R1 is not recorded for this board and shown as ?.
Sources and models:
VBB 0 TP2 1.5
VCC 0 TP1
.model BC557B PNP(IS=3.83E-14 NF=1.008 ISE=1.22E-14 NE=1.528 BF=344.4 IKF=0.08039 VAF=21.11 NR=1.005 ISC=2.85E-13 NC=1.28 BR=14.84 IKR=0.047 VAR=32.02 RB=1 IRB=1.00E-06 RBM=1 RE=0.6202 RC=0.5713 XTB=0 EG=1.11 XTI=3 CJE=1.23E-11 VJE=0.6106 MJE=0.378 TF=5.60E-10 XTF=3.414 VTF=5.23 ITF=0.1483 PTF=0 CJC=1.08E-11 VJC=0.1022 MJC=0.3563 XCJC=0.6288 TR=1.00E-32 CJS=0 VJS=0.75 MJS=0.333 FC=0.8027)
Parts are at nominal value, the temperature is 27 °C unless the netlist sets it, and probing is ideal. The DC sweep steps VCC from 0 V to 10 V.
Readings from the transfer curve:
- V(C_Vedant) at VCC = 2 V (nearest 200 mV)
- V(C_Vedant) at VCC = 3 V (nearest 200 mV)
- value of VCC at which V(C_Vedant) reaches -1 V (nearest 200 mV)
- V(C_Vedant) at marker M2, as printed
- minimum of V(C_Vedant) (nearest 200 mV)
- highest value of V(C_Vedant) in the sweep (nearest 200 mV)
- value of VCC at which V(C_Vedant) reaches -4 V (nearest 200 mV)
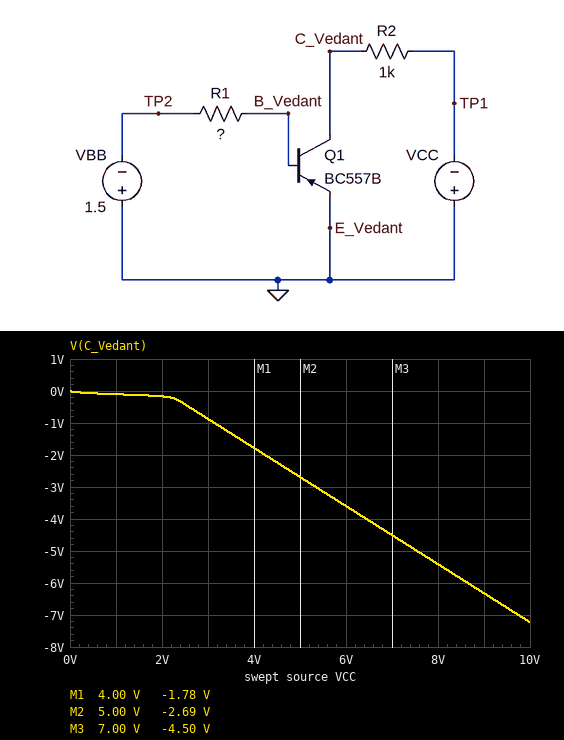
-200 mV
-800 mV
3.2 V
-2.69 V
-7.2 V
0 V
6.4 V
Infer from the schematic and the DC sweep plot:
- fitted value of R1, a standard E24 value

130 kΩ
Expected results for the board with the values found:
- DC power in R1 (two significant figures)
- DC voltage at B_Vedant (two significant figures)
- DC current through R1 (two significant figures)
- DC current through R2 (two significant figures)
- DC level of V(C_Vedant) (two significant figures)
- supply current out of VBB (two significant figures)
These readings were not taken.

7.0 µW
-550 mV
7.3 µA
3.6 µA
-3.6 mV
7.3 µA
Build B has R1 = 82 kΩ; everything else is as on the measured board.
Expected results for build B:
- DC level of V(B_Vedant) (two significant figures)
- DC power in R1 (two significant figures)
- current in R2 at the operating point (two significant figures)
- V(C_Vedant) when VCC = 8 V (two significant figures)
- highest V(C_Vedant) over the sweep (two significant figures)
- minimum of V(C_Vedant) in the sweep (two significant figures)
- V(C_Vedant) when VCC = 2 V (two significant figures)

-560 mV
11 µW
4.0 µA
-4.2 V
-4.0 mV
-5.9 V
-120 mV
